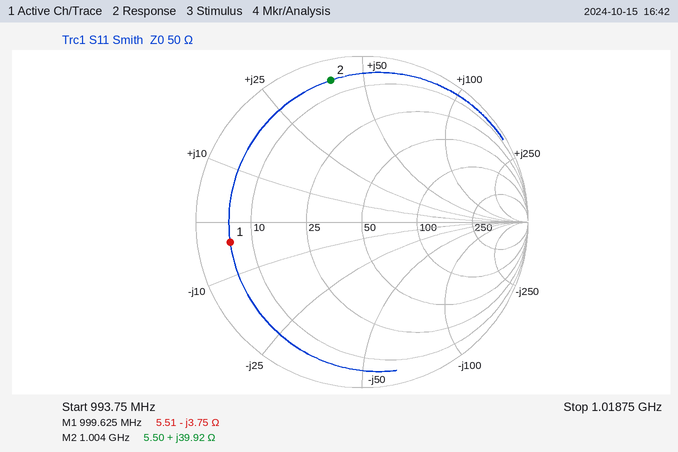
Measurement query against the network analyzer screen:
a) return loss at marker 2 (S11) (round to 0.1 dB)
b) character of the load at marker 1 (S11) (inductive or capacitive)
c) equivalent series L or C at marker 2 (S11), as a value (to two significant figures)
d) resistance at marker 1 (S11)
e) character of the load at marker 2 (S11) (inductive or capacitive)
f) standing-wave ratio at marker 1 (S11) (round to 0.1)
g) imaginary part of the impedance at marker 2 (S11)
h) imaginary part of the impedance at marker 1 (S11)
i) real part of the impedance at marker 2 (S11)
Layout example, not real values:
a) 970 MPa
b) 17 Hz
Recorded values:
a) 1.2 dB
b) capacitive
c) 6.3 nH
d) 5.51 Ω
e) inductive
f) 9.1
g) +39.92 Ω
h) -3.75 Ω
i) 5.50 Ω
